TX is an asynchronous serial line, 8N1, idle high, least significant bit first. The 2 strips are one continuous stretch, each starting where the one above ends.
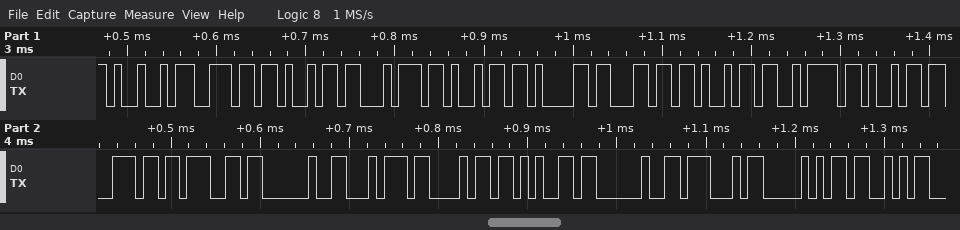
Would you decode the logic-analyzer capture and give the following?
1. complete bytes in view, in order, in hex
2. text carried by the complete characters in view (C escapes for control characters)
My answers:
49 6E 69 74 69 61 6C 69 7A 69 6E 67 20 74 68 65 20 47 50 53
"Initializing the GPS"
